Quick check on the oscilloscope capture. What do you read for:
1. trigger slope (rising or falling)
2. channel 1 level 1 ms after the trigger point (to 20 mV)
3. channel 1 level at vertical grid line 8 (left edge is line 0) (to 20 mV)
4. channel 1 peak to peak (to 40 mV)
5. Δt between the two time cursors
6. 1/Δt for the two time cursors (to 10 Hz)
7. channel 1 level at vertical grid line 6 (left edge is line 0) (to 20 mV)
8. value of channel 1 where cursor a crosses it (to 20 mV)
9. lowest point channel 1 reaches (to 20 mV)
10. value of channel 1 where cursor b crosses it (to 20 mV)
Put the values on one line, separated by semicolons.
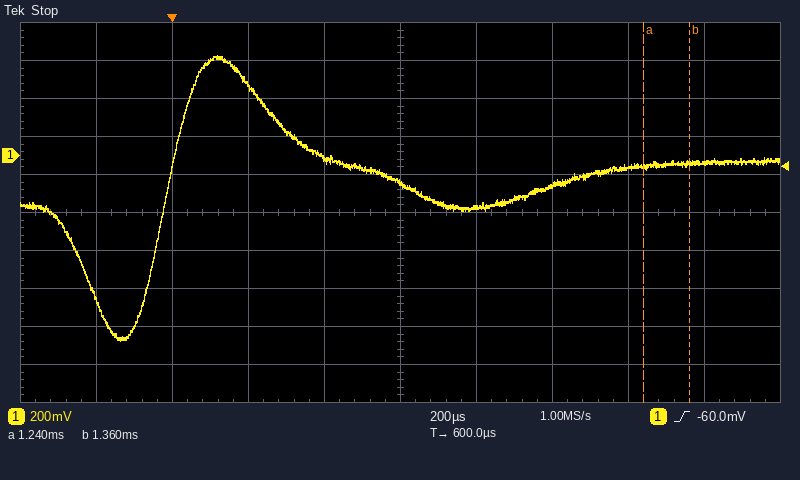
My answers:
rising; -160 mV; -60 mV; 1.52 V; 120 µs; 8.33 kHz; -280 mV; -60 mV; -980 mV; -40 mV
